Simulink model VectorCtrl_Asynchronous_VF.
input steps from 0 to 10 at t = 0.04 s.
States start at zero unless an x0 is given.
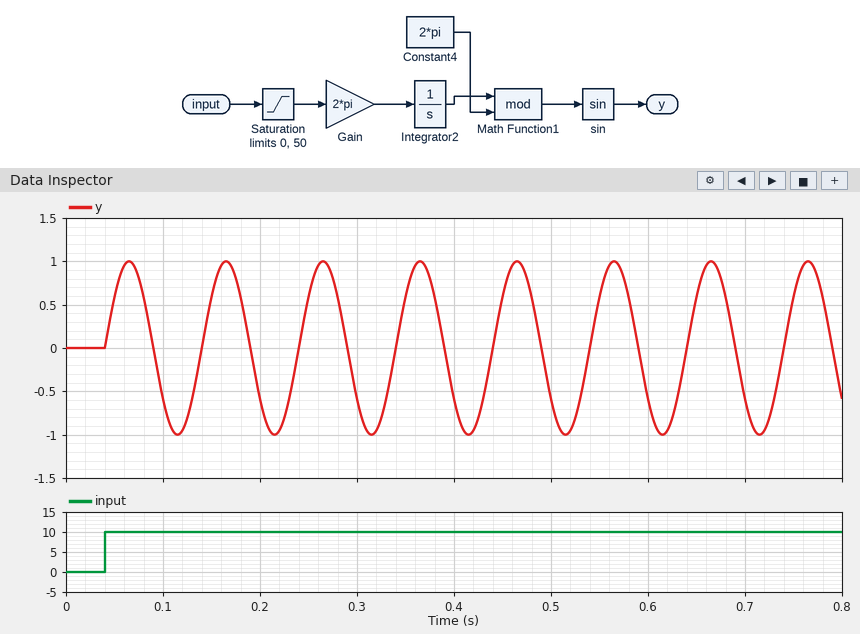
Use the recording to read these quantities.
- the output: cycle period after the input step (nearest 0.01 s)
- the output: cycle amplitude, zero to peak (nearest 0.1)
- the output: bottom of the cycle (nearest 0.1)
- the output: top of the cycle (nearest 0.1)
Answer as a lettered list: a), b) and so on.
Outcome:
a) 0.10 s
b) 1.0
c) -1.0
d) 1.0
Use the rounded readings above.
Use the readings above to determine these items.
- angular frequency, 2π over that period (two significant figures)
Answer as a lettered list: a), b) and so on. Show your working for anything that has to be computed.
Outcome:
a) 2π / 0.1 = 63 rad/s
